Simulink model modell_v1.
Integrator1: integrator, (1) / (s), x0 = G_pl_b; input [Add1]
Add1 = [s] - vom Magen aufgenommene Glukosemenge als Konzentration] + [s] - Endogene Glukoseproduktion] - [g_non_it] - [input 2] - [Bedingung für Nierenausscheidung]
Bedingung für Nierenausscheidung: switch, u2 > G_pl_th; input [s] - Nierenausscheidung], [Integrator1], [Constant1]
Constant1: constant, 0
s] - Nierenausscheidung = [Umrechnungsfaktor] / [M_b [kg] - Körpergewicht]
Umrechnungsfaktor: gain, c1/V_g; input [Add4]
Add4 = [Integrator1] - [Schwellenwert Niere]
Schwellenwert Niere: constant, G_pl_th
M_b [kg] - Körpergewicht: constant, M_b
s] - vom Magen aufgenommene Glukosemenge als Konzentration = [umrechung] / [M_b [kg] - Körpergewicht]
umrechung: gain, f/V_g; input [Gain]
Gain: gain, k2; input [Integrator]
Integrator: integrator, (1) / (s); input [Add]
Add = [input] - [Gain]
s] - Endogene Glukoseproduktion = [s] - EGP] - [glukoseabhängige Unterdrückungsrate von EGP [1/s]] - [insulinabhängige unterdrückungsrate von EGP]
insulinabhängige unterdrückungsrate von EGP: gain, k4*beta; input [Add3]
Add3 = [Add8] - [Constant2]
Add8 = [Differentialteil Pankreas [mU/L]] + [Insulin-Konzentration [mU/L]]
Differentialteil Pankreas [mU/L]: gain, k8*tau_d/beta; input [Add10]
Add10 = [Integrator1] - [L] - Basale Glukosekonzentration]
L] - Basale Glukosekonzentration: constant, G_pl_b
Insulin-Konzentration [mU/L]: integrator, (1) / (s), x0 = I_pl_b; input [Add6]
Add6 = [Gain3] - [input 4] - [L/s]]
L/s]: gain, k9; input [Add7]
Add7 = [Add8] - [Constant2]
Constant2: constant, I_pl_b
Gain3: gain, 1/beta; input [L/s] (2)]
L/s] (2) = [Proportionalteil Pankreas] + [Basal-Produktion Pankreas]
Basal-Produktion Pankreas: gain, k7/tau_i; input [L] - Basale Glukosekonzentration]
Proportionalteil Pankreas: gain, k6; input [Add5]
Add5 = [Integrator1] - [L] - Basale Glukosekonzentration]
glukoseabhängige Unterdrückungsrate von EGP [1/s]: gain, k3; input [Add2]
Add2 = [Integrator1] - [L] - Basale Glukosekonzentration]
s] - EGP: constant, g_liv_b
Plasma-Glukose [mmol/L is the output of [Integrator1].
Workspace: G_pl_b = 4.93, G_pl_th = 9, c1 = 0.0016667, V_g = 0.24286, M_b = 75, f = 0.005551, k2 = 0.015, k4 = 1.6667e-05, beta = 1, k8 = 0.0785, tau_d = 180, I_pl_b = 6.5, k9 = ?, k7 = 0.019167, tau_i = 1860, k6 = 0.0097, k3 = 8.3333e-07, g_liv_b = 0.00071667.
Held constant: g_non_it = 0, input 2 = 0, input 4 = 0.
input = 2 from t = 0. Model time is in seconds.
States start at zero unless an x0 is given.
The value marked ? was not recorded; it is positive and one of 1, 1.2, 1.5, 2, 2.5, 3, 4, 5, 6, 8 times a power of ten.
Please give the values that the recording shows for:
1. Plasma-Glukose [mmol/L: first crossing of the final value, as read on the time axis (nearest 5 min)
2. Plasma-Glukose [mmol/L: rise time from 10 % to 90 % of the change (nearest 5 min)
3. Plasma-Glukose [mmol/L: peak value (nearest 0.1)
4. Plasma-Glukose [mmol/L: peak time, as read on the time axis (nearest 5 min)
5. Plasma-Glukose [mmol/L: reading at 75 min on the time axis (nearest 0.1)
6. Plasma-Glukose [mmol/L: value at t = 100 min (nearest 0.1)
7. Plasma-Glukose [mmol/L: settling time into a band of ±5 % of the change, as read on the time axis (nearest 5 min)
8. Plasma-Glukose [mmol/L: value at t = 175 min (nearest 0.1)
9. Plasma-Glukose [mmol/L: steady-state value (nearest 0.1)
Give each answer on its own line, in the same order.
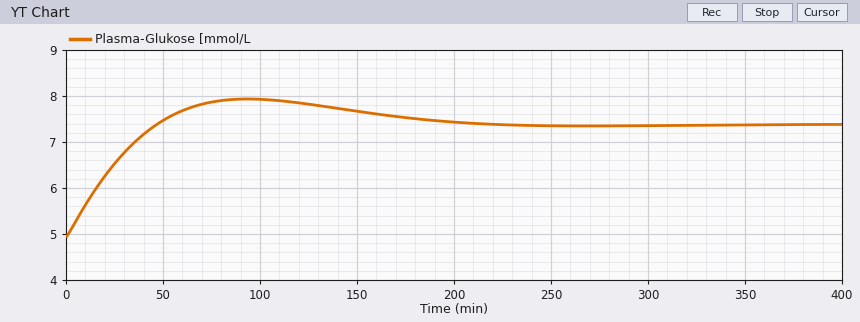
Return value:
45 min
35 min
7.9
95 min
7.9
7.9
180 min
7.5
7.4
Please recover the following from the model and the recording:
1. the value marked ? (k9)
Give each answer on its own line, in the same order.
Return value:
0.0003
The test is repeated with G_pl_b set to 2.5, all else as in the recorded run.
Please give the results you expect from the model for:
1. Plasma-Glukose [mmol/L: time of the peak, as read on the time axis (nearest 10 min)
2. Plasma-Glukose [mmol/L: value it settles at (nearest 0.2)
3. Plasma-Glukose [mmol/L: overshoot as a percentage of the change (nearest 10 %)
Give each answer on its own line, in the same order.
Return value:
90 min
5.0
20 %
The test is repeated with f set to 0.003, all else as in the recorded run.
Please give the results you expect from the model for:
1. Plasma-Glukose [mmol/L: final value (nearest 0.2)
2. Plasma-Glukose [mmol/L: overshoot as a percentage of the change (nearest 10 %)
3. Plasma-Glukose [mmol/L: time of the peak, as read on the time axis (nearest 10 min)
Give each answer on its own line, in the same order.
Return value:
6.8
20 %
90 min
